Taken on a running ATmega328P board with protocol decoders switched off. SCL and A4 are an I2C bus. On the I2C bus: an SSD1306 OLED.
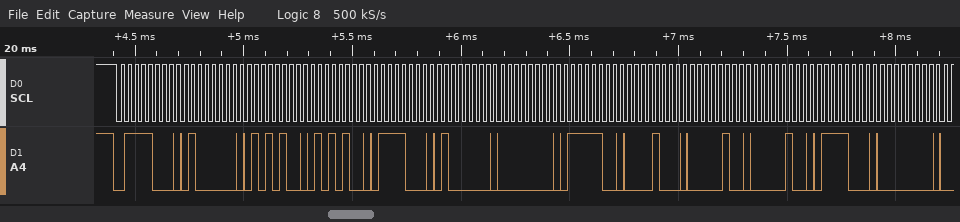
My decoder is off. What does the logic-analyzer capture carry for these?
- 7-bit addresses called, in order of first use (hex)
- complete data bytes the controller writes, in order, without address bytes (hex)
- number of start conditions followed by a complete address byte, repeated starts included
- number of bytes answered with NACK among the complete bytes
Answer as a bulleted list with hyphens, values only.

- 0x3C
- 40 54 54 78 40 00 7C 08 04 04 78 00
- 1
- 0
